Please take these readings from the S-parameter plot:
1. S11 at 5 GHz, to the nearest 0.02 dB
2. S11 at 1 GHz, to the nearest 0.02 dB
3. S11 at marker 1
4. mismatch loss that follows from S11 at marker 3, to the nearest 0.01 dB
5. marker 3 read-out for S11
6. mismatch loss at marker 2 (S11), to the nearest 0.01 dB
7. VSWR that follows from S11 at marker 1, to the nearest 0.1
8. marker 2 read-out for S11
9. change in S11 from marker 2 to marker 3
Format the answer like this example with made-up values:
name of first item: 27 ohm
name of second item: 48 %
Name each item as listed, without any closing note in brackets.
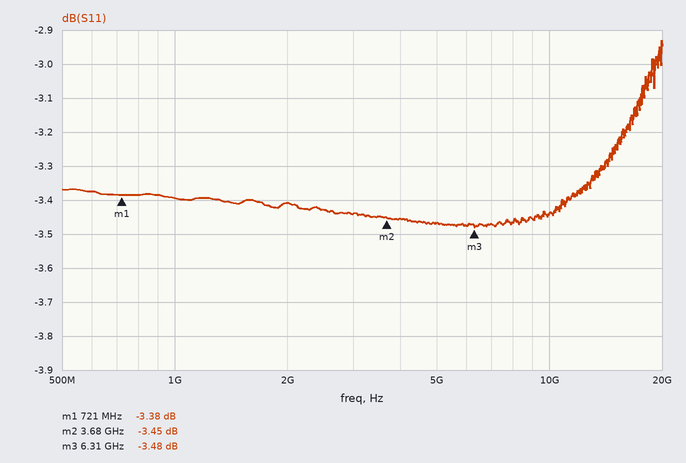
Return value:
S11 at 5 GHz, to the nearest 0.02 dB: -3.46 dB
S11 at 1 GHz, to the nearest 0.02 dB: -3.40 dB
S11 at marker 1: -3.38 dB
mismatch loss that follows from S11 at marker 3, to the nearest 0.01 dB: 2.59 dB
marker 3 read-out for S11: -3.48 dB
mismatch loss at marker 2 (S11), to the nearest 0.01 dB: 2.61 dB
VSWR that follows from S11 at marker 1, to the nearest 0.1: 5.2
marker 2 read-out for S11: -3.45 dB
change in S11 from marker 2 to marker 3: -0.03 dB
